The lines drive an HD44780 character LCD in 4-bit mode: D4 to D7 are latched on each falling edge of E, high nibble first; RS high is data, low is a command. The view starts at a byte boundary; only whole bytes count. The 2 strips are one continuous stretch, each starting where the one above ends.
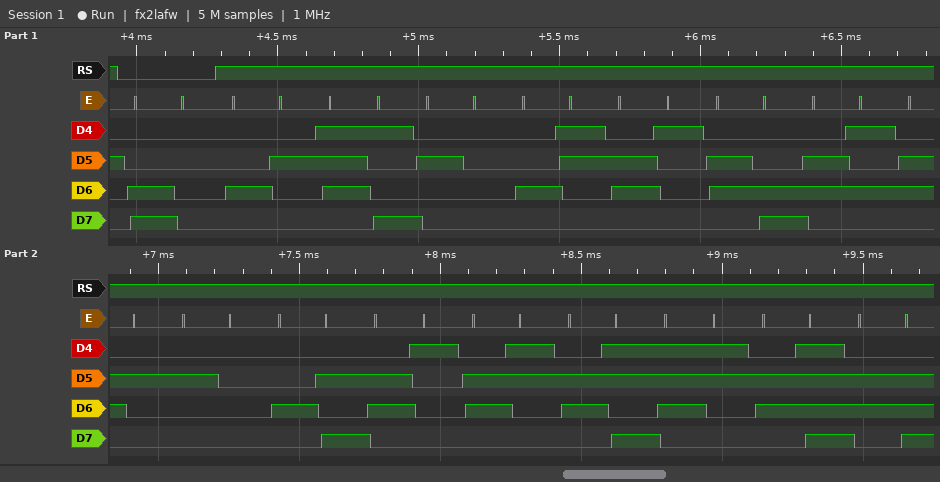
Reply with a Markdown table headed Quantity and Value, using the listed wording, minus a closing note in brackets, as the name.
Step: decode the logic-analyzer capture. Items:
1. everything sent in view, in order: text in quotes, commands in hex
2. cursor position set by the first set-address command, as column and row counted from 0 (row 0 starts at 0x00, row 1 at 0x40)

| Quantity | Value |
|---|---|
| everything sent in view, in order: text in quotes, commands in hex | 0xC0 "By Caleb Jackson" |
| cursor position set by the first set-address command, as column and row counted from 0 | column 0, row 1 |
